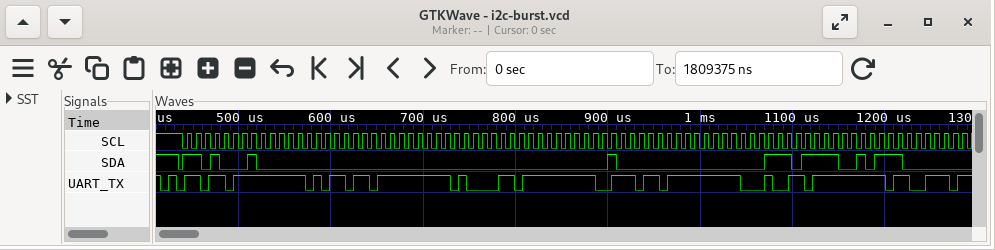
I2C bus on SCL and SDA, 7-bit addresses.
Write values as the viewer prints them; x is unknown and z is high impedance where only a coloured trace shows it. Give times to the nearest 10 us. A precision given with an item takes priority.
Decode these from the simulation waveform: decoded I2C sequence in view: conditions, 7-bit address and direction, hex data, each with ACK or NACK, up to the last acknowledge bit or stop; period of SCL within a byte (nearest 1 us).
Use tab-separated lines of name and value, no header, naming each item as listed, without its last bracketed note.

decoded I2C sequence in view: conditions, 7-bit address and direction, hex data, each with ACK or NACK, up to the last acknowledge bit or stop	start, address 68 read ACK, 00 ACK, 00 ACK, 00 ACK, 00 ACK, 40 ACK, 00 ACK, EF ACK, 5C ACK
period of SCL within a byte	10 us
